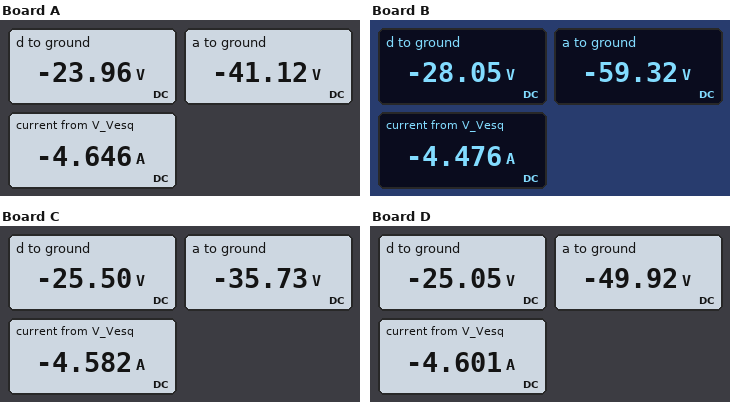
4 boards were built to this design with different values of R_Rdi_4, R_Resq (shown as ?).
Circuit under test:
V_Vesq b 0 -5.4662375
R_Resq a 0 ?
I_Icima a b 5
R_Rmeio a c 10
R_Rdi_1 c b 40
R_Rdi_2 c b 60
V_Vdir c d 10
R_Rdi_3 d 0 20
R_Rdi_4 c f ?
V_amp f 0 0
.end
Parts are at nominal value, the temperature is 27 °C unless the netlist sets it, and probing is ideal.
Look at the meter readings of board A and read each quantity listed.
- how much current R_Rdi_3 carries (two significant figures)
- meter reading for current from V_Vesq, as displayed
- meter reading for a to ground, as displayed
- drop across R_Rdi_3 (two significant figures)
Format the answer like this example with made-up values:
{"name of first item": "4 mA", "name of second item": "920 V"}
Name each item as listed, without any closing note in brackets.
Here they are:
{"how much current R_Rdi_3 carries": "1.2 A", "meter reading for current from V_Vesq, as displayed": "-4.646 A", "meter reading for a to ground, as displayed": "-41.12 V", "drop across R_Rdi_3": "24 V"}
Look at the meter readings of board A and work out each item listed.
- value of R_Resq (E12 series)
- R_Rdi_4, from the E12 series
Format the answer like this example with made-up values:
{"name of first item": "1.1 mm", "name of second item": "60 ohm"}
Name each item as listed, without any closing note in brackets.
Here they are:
{"value of R_Resq": "18 Ω", "R_Rdi_4, from the E12 series": "12 Ω"}
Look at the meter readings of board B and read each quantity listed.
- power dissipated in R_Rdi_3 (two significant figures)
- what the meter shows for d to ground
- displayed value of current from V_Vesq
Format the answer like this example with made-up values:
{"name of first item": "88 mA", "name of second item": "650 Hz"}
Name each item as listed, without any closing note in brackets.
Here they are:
{"power dissipated in R_Rdi_3": "39 W", "what the meter shows for d to ground": "-28.05 V", "displayed value of current from V_Vesq": "-4.476 A"}
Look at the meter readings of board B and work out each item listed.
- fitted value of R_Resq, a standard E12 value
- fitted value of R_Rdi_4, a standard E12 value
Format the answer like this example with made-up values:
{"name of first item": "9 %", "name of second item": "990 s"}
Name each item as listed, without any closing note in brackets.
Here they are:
{"fitted value of R_Resq, a standard E12 value": "68 Ω", "fitted value of R_Rdi_4, a standard E12 value": "8.2 Ω"}
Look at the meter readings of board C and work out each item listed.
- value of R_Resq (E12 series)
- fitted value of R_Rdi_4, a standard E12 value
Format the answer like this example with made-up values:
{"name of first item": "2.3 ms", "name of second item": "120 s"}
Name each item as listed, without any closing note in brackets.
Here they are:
{"value of R_Resq": "12 Ω", "fitted value of R_Rdi_4, a standard E12 value": "47 Ω"}
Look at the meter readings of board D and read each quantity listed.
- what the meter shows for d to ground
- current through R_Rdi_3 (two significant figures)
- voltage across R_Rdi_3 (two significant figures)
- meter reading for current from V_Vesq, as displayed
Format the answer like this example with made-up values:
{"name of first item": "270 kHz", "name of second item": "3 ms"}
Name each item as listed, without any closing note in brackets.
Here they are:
{"what the meter shows for d to ground": "-25.05 V", "current through R_Rdi_3": "1.3 A", "voltage across R_Rdi_3": "25 V", "meter reading for current from V_Vesq, as displayed": "-4.601 A"}
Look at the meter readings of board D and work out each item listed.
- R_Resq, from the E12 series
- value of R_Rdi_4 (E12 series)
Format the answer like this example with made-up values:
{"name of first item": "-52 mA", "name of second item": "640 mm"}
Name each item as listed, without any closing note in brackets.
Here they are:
{"R_Resq, from the E12 series": "33 Ω", "value of R_Rdi_4": "8.2 Ω"}
